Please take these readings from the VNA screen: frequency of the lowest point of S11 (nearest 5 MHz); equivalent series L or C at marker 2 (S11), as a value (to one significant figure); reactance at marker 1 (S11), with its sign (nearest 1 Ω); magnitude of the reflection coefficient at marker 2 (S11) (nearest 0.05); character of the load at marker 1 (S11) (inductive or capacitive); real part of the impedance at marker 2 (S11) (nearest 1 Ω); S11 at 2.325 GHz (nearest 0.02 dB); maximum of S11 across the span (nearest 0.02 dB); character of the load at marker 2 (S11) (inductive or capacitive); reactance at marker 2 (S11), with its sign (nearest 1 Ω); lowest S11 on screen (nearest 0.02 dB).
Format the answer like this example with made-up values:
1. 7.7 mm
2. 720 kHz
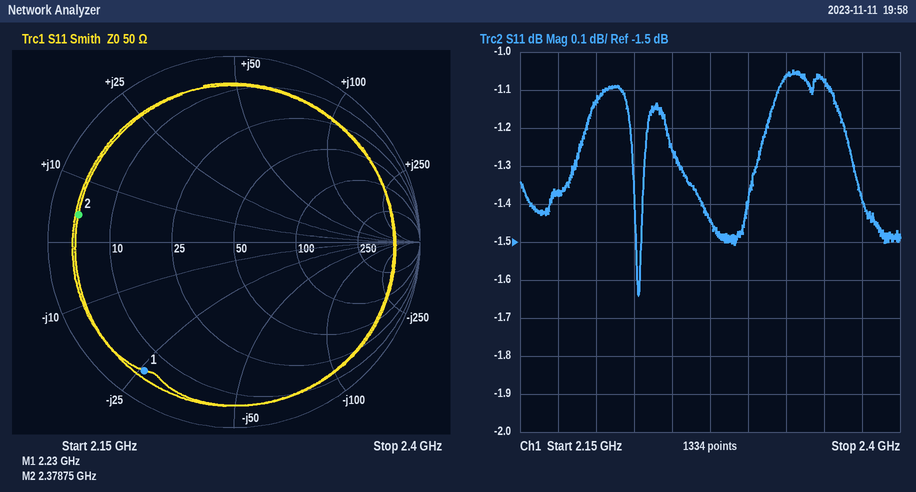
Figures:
1. 2.230 GHz
2. 300 pH
3. -26 Ω
4. 0.85
5. capacitive
6. 4 Ω
7. -1.06 dB
8. -1.04 dB
9. inductive
10. +4 Ω
11. -1.64 dB
